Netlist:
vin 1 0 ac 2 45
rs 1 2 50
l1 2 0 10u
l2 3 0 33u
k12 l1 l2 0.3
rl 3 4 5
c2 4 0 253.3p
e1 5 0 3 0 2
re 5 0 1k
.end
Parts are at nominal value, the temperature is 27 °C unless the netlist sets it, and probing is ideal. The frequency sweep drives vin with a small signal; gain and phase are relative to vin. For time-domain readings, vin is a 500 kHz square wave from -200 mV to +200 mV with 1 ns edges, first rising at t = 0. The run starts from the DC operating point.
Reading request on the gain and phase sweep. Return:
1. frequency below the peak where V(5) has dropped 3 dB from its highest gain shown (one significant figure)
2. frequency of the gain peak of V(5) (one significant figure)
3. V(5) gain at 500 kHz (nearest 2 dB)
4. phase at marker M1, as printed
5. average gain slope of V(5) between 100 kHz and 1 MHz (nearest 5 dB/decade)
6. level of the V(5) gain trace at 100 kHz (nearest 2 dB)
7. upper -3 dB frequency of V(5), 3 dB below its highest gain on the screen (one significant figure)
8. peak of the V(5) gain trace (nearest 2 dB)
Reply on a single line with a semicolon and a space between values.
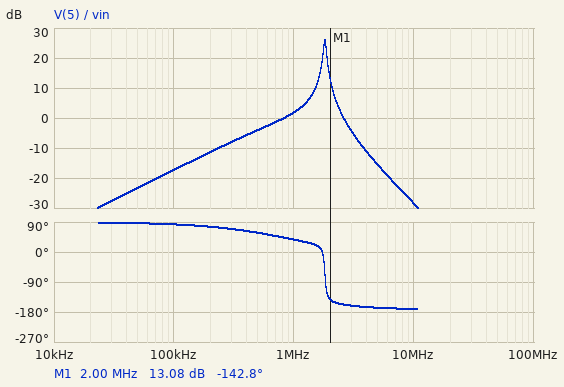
2 MHz; 2 MHz; -4 dB; -142.8 deg; 20 dB/decade; -18 dB; 2 MHz; 26 dB
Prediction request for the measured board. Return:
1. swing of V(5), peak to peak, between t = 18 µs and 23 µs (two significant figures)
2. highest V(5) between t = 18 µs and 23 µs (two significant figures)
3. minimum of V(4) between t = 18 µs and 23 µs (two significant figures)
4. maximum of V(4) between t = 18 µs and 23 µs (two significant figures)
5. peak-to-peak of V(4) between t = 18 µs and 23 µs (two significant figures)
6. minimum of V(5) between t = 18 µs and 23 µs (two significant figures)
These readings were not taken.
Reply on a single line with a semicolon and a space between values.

830 mV; 410 mV; -210 mV; 210 mV; 410 mV; -410 mV
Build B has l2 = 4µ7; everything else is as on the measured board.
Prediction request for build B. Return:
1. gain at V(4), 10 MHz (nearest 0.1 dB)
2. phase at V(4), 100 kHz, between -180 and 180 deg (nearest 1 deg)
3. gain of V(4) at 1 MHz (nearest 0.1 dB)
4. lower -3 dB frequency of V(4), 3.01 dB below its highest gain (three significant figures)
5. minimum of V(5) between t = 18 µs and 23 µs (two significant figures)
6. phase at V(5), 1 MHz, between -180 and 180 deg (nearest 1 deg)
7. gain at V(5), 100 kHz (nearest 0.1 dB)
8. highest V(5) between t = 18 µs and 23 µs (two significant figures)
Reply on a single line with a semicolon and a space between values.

-24.1 dB; 83 deg; -15.5 dB; 4.69 MHz; -230 mV; 38 deg; -25.8 dB; 230 mV
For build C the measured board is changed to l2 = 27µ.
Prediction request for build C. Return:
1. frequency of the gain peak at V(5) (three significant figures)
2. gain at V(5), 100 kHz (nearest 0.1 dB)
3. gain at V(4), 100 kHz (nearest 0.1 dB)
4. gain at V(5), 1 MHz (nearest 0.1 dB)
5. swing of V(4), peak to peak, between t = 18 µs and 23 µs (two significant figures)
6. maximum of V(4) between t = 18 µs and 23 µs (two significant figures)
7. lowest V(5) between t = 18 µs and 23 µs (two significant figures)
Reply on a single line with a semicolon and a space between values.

2.00 MHz; -18.2 dB; -24.2 dB; 0.3 dB; 320 mV; 160 mV; -320 mV
